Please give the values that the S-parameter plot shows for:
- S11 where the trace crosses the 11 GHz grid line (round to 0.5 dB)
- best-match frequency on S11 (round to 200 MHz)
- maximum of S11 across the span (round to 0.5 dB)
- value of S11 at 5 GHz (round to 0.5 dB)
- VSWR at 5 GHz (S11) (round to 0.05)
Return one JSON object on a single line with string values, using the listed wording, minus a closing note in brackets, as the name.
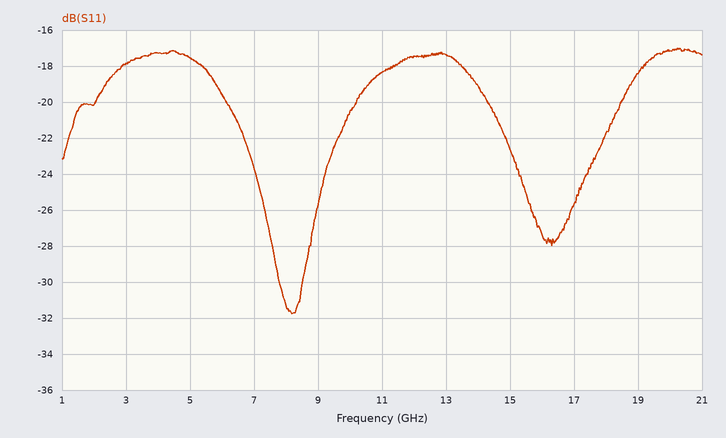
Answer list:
{"S11 where the trace crosses the 11 GHz grid line": "-18.5 dB", "best-match frequency on S11": "8.2 GHz", "maximum of S11 across the span": "-17.0 dB", "value of S11 at 5 GHz": "-17.5 dB", "VSWR at 5 GHz (S11)": "1.30"}
